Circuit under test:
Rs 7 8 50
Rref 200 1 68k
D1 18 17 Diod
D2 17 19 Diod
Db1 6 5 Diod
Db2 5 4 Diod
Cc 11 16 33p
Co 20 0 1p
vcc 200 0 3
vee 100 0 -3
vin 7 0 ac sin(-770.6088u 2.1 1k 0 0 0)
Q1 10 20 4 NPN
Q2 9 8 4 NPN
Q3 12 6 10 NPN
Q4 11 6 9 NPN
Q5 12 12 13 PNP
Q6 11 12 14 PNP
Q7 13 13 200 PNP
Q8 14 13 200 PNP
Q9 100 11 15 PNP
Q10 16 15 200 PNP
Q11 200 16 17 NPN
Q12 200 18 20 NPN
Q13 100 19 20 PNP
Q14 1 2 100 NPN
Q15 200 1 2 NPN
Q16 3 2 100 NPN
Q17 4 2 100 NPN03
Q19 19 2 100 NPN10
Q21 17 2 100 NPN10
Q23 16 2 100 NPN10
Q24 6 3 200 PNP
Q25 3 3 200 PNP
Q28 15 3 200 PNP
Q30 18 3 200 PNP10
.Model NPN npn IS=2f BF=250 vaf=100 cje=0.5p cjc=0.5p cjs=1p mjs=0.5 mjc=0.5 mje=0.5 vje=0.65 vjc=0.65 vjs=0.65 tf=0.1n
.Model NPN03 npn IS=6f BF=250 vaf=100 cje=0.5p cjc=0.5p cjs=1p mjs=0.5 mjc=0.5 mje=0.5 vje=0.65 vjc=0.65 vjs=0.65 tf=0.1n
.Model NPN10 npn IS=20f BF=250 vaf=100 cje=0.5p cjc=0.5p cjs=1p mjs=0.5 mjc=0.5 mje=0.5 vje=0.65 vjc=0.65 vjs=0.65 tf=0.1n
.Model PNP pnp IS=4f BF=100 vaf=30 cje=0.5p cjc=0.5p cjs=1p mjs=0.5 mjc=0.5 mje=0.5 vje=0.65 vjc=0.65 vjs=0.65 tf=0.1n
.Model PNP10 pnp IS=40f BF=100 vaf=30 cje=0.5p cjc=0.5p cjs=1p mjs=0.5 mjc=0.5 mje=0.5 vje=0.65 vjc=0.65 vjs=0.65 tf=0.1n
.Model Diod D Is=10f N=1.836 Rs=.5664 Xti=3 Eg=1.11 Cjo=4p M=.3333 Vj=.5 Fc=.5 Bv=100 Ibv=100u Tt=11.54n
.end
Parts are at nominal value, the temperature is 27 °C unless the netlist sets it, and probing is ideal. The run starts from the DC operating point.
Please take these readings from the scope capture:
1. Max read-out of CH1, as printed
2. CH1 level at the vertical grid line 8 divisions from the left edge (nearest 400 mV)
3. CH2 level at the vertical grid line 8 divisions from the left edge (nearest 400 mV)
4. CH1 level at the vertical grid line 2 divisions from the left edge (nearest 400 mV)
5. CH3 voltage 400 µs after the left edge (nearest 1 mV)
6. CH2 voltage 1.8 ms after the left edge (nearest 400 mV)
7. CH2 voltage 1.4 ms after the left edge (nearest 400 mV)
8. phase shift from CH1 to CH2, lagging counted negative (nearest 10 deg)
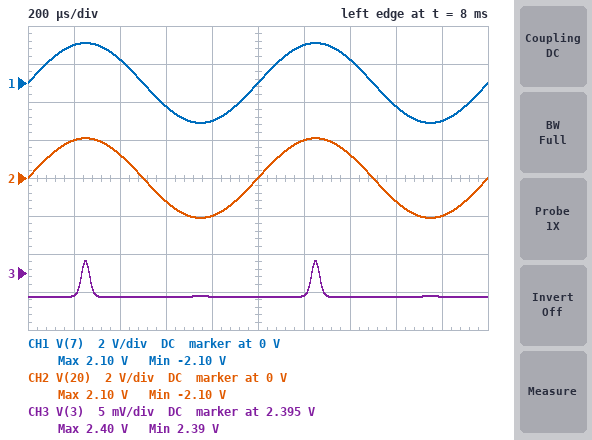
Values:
2.10 V
-1.2 V
-1.2 V
1.2 V
2.392 V
-2.0 V
1.2 V
0 deg
